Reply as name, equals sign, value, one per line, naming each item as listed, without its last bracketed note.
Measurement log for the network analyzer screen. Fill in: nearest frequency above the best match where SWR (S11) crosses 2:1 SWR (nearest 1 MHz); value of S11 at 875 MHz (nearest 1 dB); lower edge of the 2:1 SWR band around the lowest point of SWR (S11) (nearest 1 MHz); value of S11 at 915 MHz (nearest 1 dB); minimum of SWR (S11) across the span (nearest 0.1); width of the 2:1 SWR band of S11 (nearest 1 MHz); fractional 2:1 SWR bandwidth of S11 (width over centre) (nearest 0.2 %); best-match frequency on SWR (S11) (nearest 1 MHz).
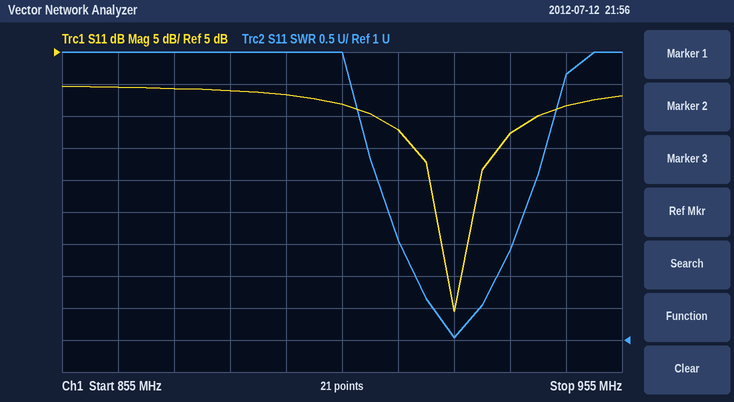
nearest frequency above the best match where SWR (S11) crosses 2:1 SWR = 933 MHz
value of S11 at 875 MHz = -1 dB
lower edge of the 2:1 SWR band around the lowest point of SWR (S11) = 918 MHz
value of S11 at 915 MHz = -7 dB
minimum of SWR (S11) across the span = 1.0
width of the 2:1 SWR band of S11 = 15 MHz
fractional 2:1 SWR bandwidth of S11 (width over centre) = 1.6 %
best-match frequency on SWR (S11) = 925 MHz
